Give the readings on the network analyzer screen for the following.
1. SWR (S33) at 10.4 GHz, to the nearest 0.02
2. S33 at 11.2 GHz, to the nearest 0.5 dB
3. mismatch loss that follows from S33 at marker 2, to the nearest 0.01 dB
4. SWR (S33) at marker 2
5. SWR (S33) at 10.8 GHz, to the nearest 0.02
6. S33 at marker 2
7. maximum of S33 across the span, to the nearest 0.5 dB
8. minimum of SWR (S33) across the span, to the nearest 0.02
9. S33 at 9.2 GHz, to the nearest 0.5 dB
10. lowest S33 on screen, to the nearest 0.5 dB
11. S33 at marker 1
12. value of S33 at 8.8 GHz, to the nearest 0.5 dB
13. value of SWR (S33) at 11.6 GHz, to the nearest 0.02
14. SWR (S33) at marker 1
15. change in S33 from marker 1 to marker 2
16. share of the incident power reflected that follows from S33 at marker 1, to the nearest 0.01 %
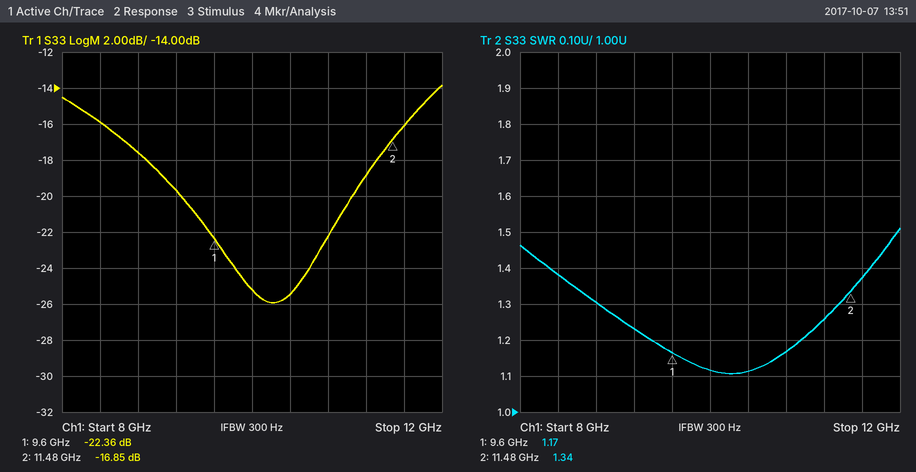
1.12
-19.0 dB
0.09 dB
1.34
1.16
-16.85 dB
-14.0 dB
1.10
-19.5 dB
-26.0 dB
-22.36 dB
-17.5 dB
1.38
1.17
5.51 dB
0.58 %
